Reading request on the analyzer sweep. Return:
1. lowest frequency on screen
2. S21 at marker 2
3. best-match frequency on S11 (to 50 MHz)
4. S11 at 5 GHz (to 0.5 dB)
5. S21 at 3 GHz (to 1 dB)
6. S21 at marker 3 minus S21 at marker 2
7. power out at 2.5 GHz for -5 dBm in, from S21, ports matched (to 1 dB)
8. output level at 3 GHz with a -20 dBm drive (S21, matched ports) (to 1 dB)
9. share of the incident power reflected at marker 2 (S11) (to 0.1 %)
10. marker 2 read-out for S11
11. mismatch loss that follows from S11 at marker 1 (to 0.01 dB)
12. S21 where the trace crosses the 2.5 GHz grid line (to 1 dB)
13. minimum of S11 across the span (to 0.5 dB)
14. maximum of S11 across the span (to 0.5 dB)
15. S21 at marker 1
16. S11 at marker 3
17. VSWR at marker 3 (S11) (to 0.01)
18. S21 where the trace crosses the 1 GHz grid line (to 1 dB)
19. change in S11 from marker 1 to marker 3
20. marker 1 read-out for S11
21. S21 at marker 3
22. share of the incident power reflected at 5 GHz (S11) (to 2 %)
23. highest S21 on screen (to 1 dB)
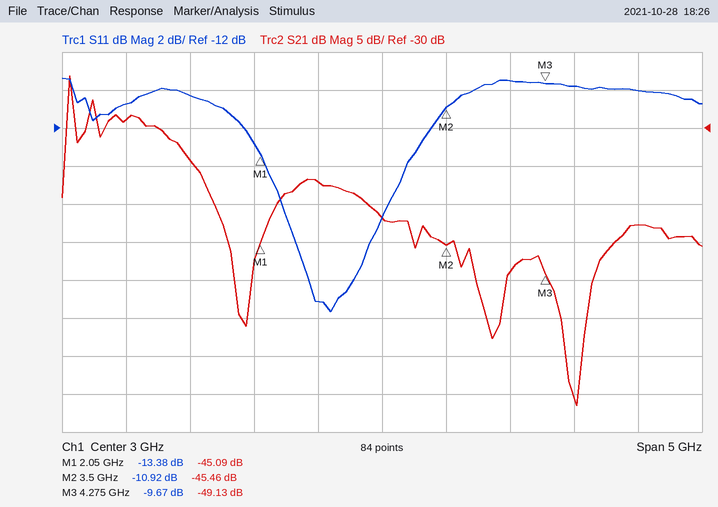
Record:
500 MHz
-45.46 dB
2.60 GHz
-10.0 dB
-42 dB
-3.67 dB
-42 dBm
-62 dBm
8.1 %
-10.92 dB
0.20 dB
-37 dB
-21.5 dB
-9.5 dB
-45.09 dB
-9.67 dB
1.98
-29 dB
3.71 dB
-13.38 dB
-49.13 dB
10 %
-23 dB
